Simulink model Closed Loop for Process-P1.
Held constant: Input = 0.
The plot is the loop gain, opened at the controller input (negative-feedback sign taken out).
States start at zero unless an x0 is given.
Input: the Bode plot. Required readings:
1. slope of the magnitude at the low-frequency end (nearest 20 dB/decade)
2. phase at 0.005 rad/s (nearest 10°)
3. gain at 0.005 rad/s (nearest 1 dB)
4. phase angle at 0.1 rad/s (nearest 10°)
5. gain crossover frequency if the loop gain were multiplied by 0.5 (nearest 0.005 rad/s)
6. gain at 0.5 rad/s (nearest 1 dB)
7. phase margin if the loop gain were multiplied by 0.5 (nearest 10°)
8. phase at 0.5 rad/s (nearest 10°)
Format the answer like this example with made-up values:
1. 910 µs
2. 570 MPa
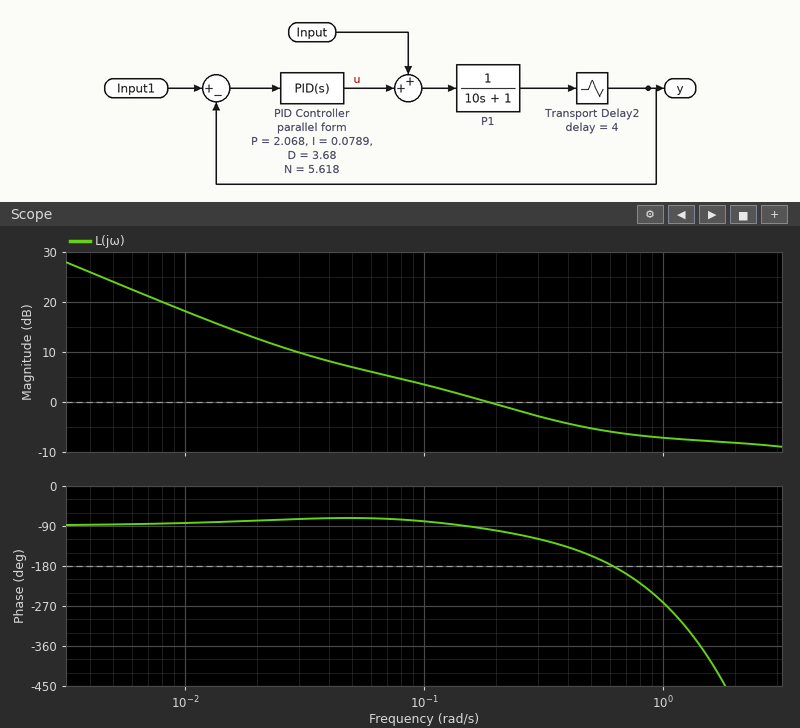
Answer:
1. -20 dB/decade
2. -90°
3. 24 dB
4. -80°
5. 0.060 rad/s
6. -5 dB
7. 110°
8. -160°
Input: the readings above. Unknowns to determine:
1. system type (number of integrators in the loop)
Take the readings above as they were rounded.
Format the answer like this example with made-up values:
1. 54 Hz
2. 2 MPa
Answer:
1. 1
